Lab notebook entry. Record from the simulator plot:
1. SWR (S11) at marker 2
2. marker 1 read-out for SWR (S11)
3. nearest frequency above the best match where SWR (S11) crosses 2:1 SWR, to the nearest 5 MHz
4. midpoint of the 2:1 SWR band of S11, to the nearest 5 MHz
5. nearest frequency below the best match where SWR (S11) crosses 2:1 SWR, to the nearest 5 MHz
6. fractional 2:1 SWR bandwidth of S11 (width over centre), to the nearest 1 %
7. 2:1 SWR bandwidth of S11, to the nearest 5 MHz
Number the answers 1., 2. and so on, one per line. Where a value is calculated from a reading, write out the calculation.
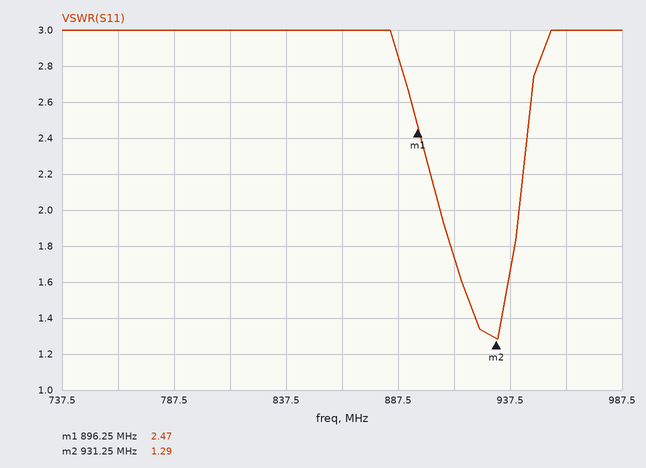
1. 1.29
2. 2.47
3. 940 MHz
4. 925 MHz
5. 905 MHz
6. 35 MHz / 922.5 MHz ≈ 4 %
7. 940 MHz − 905 MHz = 35 MHz
